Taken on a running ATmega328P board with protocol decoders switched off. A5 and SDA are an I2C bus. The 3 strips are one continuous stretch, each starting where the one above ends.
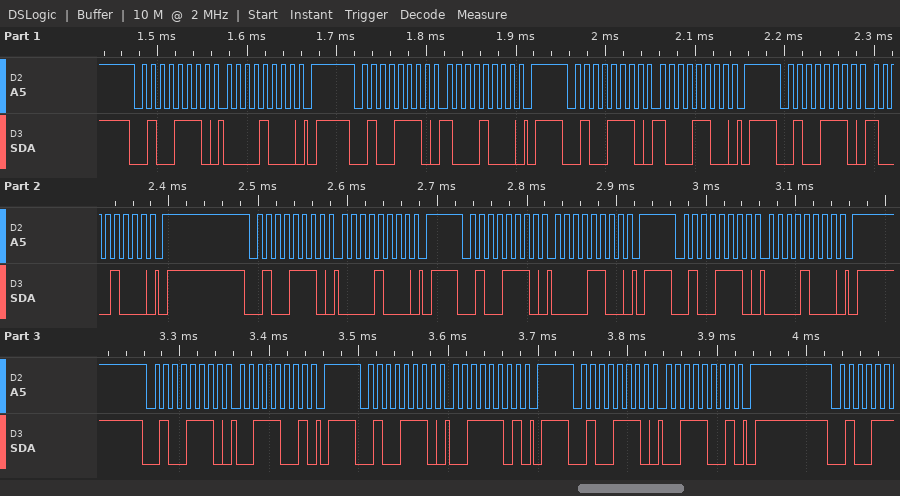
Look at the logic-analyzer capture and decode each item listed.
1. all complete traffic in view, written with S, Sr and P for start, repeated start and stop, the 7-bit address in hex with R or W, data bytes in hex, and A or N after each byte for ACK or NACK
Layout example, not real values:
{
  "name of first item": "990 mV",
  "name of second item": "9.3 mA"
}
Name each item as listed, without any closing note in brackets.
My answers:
{
  "all complete traffic in view, written with S, Sr and P for start, repeated start and stop, the 7-bit address in hex with R or W, data bytes in hex, and A or N after each byte for ACK or NACK": "S 27W A 08 A P S 27W A 88 A P S 27W A 8C A P S 27W A 88 A P S 27W A 08 A P S 27W A 0C A P S 27W A 08 A P S 27W A 39 A P S 27W A 3D A P S 27W A 39 A P"
}
